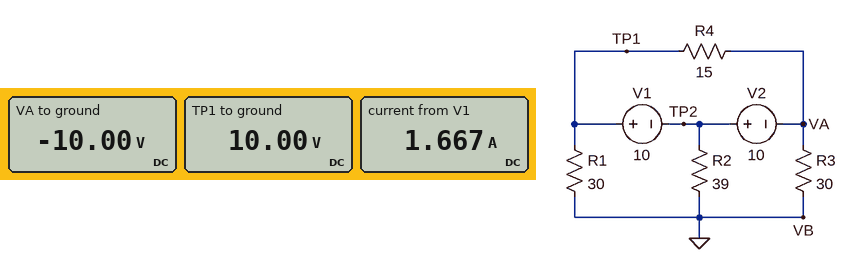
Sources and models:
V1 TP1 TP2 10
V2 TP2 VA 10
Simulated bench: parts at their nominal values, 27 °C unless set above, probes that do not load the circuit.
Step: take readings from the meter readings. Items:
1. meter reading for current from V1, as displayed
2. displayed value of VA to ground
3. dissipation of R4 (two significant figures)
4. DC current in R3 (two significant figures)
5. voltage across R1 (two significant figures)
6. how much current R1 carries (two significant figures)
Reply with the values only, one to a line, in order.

1.667 A
-10.00 V
27 W
330 mA
10 V
330 mA
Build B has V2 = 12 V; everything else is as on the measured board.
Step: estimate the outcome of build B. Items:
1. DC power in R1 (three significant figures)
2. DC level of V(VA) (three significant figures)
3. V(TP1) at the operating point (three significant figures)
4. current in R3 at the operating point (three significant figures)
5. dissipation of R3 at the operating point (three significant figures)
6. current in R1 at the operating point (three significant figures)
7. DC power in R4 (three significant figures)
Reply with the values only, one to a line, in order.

3.83 W
-11.3 V
10.7 V
376 mA
4.24 W
357 mA
32.3 W
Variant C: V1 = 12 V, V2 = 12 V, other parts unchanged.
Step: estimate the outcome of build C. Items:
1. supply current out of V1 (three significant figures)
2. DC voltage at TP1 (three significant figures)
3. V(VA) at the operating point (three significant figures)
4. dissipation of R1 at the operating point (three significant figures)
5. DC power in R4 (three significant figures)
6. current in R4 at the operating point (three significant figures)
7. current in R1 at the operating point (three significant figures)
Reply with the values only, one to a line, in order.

2.00 A
12.0 V
-12.0 V
4.80 W
38.4 W
1.60 A
400 mA
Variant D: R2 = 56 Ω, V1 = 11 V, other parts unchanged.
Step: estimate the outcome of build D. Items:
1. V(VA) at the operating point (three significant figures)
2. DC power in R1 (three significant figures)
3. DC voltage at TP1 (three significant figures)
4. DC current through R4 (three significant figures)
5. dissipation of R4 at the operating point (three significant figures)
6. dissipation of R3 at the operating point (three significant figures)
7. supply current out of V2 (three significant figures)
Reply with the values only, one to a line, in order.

-10.4 V
3.75 W
10.6 V
1.40 A
29.4 W
3.60 W
1.75 A
